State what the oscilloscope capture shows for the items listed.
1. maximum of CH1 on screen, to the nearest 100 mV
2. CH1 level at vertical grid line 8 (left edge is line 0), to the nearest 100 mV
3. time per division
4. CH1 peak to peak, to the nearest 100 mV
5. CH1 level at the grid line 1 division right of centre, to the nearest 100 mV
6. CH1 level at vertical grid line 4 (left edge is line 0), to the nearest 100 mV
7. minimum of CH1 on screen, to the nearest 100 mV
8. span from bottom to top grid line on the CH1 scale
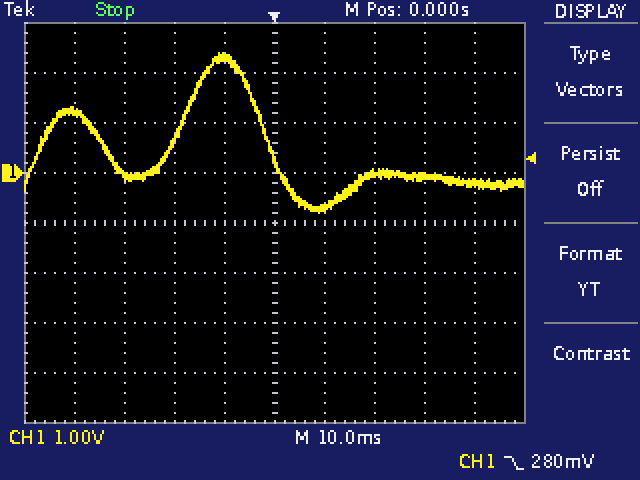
2.4 V
-100 mV
10 ms
3.2 V
-700 mV
2.3 V
-800 mV
8 V
